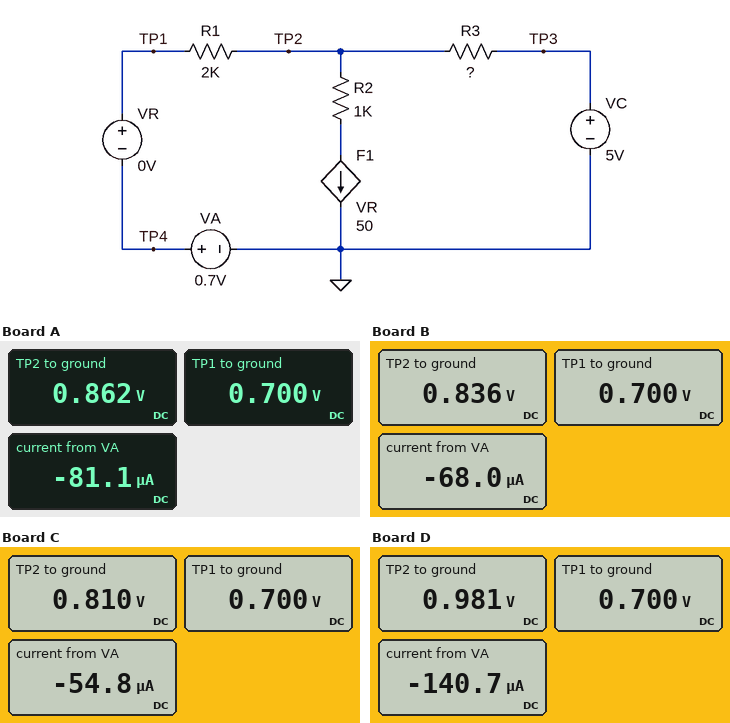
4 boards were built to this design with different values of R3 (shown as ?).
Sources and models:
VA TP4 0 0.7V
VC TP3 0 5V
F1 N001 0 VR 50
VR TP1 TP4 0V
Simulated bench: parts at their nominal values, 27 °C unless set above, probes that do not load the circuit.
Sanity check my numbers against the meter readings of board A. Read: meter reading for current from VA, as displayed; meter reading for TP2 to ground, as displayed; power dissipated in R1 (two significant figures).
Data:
-81.1 µA
0.862 V
13 µW
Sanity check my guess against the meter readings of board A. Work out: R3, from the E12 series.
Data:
1 kΩ
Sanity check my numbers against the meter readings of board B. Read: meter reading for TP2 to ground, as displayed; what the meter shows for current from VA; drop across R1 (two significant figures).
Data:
0.836 V
-68.0 µA
140 mV
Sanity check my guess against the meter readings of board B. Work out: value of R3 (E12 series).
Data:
1.2 kΩ
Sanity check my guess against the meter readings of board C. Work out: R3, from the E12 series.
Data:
1.5 kΩ
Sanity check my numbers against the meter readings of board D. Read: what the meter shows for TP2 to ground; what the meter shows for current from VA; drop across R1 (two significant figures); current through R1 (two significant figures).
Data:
0.981 V
-140.7 µA
280 mV
140 µA
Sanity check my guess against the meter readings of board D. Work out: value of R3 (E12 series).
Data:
560 Ω
